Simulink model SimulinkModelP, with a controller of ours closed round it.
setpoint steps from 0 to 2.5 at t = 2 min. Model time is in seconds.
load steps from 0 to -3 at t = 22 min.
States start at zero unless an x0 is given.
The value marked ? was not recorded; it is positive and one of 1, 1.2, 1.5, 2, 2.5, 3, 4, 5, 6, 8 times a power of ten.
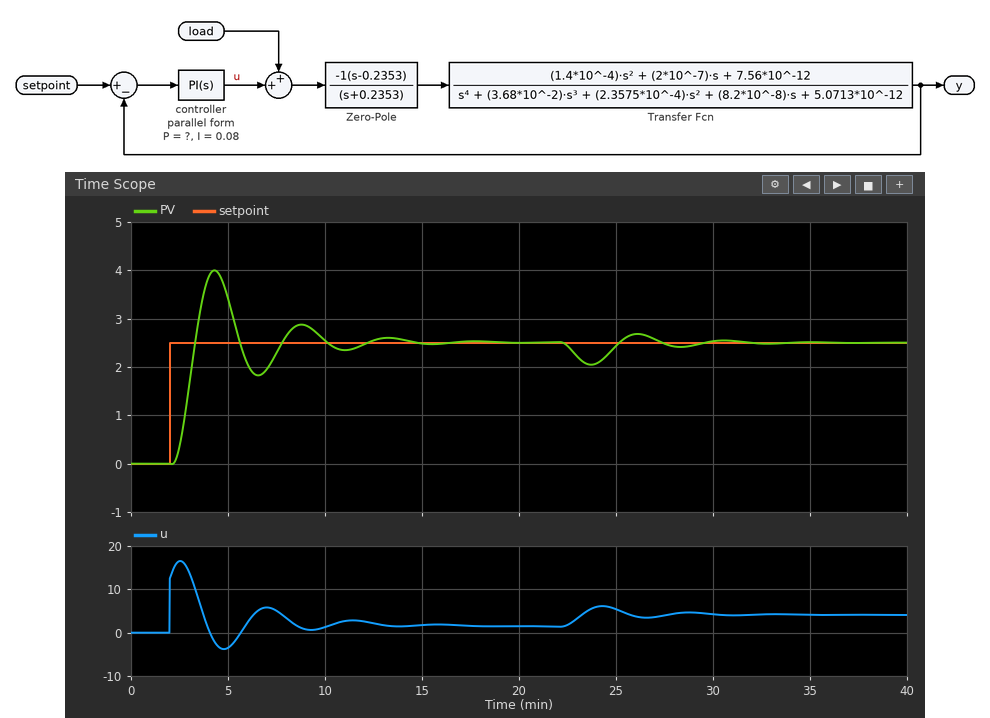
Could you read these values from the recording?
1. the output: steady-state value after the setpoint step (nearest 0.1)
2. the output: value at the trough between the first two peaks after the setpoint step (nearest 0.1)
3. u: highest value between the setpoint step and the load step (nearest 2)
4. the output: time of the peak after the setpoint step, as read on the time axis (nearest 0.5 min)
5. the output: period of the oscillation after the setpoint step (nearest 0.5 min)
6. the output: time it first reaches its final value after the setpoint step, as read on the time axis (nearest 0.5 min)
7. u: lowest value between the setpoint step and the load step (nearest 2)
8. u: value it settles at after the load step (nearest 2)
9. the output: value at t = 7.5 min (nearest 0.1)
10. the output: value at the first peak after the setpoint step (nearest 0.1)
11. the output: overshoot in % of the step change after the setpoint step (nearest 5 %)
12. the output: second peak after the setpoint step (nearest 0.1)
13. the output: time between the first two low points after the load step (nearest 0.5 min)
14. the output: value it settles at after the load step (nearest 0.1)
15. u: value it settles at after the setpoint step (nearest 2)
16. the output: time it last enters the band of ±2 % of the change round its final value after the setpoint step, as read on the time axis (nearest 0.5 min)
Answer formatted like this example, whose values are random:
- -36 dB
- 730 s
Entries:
- 2.5
- 1.8
- 16
- 4.5 min
- 4.5 min
- 3.5 min
- -4
- 4
- 2.3
- 4.0
- 60 %
- 2.9
- 4.5 min
- 2.5
- 2
- 14.0 min
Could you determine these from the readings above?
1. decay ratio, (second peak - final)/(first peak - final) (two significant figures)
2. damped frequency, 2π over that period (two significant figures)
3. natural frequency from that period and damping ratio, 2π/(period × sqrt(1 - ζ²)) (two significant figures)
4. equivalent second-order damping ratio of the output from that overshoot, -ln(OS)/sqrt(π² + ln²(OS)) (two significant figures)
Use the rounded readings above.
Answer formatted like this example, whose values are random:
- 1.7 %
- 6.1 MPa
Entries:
- 0.27
- 1.4 rad/min
- 1.4 rad/min
- 0.16
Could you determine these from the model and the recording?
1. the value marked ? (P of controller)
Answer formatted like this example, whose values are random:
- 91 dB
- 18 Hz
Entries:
- 5
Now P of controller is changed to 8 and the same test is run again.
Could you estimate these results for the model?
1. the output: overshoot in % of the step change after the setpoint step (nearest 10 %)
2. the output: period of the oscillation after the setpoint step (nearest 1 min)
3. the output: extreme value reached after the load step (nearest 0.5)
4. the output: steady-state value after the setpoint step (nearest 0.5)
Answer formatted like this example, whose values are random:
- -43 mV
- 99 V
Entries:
- 50 %
- 3 min
- 2.0
- 2.5
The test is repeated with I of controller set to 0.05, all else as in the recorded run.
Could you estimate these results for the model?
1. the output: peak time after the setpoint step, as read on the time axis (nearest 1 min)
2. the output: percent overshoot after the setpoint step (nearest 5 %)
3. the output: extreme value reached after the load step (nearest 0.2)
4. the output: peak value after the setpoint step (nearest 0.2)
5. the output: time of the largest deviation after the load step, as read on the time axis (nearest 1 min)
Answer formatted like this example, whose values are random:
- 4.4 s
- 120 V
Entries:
- 4 min
- 40 %
- 2.0
- 3.4
- 24 min
